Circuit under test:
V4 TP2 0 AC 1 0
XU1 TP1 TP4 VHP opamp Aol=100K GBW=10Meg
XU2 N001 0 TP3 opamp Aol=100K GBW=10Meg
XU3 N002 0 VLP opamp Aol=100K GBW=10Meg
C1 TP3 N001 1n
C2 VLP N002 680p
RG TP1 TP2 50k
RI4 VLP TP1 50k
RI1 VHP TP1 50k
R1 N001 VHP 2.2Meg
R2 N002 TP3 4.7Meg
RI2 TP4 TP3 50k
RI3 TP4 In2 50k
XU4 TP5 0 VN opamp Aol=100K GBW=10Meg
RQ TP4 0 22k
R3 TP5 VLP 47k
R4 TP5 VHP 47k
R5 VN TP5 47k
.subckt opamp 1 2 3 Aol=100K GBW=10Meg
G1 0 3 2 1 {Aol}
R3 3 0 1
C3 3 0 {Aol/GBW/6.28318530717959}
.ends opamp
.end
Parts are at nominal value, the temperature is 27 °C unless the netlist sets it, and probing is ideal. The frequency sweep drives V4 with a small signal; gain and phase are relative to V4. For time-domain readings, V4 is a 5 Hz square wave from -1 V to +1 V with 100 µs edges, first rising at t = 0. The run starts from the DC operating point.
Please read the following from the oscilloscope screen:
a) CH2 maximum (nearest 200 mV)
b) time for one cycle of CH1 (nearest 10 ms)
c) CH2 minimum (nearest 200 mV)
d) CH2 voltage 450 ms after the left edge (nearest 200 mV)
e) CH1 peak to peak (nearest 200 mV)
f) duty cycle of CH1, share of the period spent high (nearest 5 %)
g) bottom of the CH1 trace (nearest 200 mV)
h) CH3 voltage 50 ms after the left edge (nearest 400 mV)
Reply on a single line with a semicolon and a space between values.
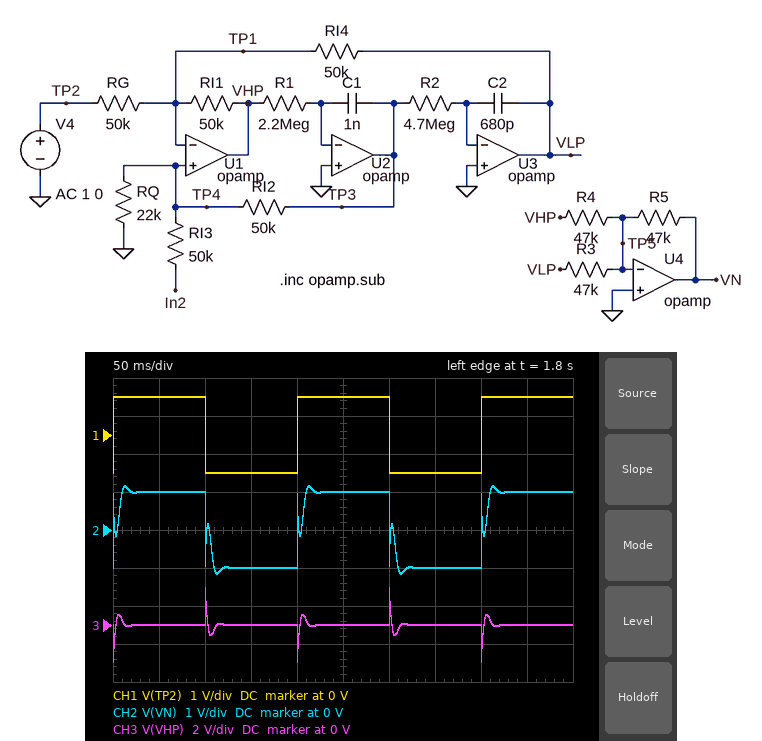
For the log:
1.2 V; 200 ms; -1.2 V; 1.0 V; 2.0 V; 50 %; -1.0 V; 0 V
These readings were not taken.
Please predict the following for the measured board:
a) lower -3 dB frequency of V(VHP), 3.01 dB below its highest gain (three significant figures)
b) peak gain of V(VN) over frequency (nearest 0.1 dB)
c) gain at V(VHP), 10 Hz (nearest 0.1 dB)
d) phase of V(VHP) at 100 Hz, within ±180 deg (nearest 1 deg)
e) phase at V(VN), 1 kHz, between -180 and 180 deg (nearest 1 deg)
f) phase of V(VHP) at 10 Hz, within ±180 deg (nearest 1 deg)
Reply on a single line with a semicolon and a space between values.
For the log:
52.4 Hz; 0 dB; -31.0 dB; -134 deg; 4 deg; -11 deg
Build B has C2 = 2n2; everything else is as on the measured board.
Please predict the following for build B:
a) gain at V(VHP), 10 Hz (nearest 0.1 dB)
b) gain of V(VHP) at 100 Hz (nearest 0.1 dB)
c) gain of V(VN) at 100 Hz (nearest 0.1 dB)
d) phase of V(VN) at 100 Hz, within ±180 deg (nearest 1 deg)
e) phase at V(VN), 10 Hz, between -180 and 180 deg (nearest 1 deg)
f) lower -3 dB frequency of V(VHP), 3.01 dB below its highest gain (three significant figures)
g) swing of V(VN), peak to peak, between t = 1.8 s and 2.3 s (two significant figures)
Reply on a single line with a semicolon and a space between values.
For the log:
-21.7 dB; -0.9 dB; -1.9 dB; 37 deg; -33 deg; 51.4 Hz; 2.0 V
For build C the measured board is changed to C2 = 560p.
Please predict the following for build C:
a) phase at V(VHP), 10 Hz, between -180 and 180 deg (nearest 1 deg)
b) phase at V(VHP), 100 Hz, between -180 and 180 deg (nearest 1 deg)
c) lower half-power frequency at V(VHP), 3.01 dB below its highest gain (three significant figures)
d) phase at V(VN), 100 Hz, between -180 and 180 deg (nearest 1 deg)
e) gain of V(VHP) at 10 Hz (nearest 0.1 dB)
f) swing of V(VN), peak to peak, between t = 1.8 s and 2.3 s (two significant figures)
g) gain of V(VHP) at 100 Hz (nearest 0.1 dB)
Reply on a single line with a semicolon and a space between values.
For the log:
-9 deg; -130 deg; 56.6 Hz; 50 deg; -32.7 dB; 2.4 V; 1.2 dB
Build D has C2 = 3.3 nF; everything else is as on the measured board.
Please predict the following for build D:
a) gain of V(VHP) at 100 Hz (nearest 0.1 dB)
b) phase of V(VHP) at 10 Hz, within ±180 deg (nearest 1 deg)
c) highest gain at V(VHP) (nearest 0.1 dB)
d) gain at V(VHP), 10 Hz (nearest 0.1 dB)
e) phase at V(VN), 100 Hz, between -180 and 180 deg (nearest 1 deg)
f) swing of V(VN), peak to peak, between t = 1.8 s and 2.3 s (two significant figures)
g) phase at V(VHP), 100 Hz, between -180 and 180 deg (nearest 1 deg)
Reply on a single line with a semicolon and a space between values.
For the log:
-1.1 dB; -46 deg; 0 dB; -19.3 dB; 36 deg; 2.0 V; -144 deg
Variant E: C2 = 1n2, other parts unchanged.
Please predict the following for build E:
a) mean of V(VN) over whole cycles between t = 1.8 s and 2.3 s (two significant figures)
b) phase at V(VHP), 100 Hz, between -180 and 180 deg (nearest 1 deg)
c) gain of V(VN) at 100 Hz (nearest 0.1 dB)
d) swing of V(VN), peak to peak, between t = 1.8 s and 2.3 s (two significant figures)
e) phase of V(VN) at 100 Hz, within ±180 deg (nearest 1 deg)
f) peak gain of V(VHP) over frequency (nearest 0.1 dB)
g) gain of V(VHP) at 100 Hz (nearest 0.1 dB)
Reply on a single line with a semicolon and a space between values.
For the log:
170 mV; -140 deg; -2.3 dB; 2.1 V; 40 deg; 0 dB; -0.3 dB
